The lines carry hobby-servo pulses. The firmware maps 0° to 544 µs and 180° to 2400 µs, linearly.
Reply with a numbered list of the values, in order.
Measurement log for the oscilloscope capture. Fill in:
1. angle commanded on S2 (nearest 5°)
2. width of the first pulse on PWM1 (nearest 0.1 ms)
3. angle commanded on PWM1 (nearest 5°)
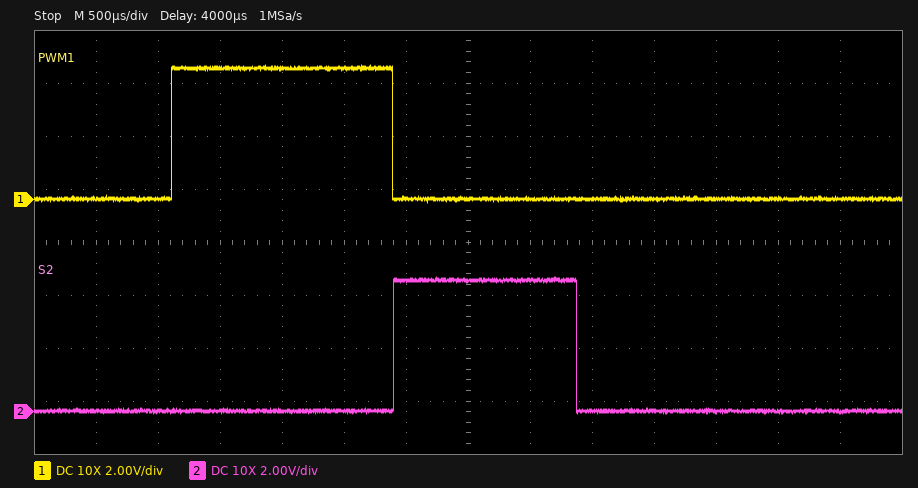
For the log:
1. 90°
2. 1.8 ms
3. 120°
